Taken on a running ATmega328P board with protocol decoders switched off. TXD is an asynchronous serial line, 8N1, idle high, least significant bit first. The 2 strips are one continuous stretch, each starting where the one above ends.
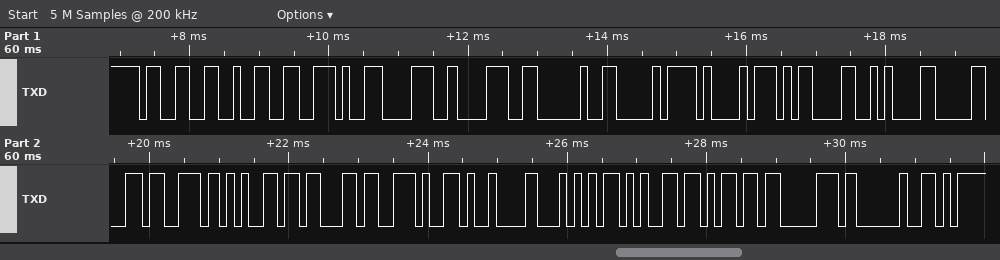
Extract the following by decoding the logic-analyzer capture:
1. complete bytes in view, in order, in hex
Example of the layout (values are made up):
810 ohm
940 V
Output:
0x33 0x32 0x2E 0x38 0x38 0x20 0xD0 0xA1 0x0D 0x0A 0x30 0x73 0x65 0x63 0x2E 0x09 0x54 0x65 0x6D 0x70 0x20
